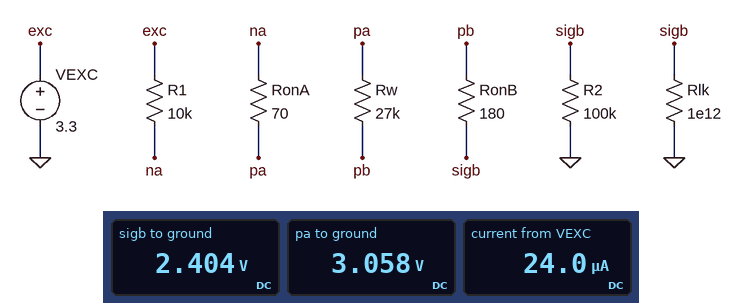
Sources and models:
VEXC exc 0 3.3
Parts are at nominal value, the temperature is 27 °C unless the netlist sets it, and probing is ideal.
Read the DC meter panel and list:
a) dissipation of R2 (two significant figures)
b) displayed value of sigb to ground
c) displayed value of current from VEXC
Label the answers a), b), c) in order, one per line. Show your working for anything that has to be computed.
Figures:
a) (2.404 V)^2 / 100 kΩ = 58 µW
b) 2.404 V
c) 24.0 µA
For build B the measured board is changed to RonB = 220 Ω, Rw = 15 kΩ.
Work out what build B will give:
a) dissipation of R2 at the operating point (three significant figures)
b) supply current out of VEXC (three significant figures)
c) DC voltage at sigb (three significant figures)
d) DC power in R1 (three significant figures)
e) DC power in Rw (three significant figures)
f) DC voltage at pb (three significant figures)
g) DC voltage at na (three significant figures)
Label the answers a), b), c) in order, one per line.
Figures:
a) 69.4 µW
b) 26.3 µA
c) 2.63 V
d) 6.94 µW
e) 10.4 µW
f) 2.64 V
g) 3.04 V
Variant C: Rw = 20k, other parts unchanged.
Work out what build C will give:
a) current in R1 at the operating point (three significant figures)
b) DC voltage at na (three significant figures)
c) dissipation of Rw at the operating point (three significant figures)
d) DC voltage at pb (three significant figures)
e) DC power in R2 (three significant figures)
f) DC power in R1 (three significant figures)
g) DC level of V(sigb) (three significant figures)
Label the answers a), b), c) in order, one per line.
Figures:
a) 25.3 µA
b) 3.05 V
c) 12.8 µW
d) 2.54 V
e) 64.2 µW
f) 6.42 µW
g) 2.53 V
